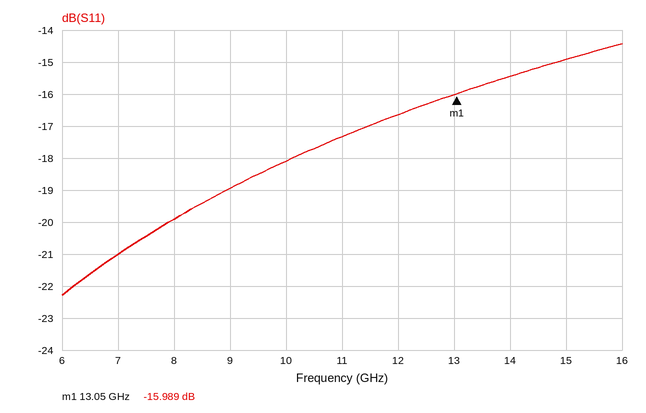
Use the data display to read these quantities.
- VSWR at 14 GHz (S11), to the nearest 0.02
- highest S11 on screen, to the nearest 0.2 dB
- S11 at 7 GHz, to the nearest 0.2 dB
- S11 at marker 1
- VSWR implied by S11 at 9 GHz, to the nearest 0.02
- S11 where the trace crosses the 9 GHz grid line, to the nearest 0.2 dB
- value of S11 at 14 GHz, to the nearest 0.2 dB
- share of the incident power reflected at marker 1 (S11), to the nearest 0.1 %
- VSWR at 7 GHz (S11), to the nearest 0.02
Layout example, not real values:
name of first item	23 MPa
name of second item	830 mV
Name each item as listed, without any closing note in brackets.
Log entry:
VSWR at 14 GHz (S11), to the nearest 0.02	1.40
highest S11 on screen, to the nearest 0.2 dB	-14.4 dB
S11 at 7 GHz, to the nearest 0.2 dB	-21.0 dB
S11 at marker 1	-15.989 dB
VSWR implied by S11 at 9 GHz, to the nearest 0.02	1.26
S11 where the trace crosses the 9 GHz grid line, to the nearest 0.2 dB	-19.0 dB
value of S11 at 14 GHz, to the nearest 0.2 dB	-15.4 dB
share of the incident power reflected at marker 1 (S11), to the nearest 0.1 %	2.5 %
VSWR at 7 GHz (S11), to the nearest 0.02	1.20
